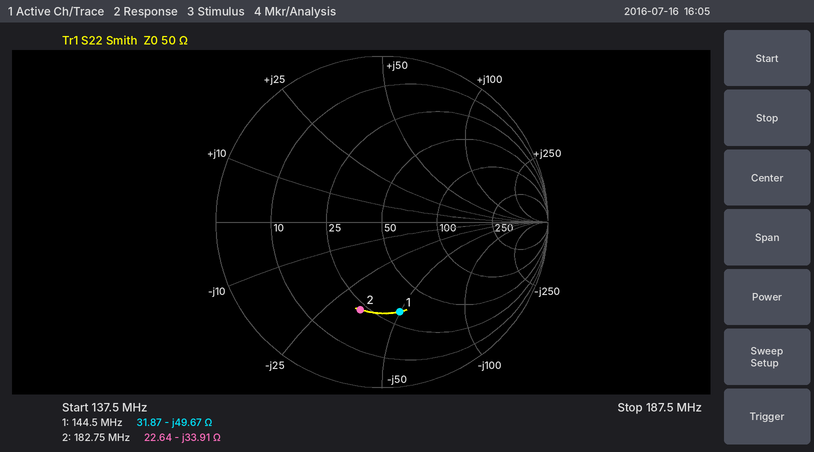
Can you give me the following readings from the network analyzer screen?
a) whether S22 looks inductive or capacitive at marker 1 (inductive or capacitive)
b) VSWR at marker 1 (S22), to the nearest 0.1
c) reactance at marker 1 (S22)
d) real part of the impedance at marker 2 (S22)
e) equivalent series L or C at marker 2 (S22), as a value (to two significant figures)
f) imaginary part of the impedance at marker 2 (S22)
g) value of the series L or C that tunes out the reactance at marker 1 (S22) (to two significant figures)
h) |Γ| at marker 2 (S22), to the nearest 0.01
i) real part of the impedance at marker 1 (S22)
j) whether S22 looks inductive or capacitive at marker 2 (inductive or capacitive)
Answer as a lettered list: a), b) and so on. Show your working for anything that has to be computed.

a) capacitive
b) 3.5
c) -49.67 Ω
d) 22.64 Ω
e) C = 1/(2π × 182.75 MHz × 33.91 Ω) ≈ 26 pF
f) -33.91 Ω
g) L = 49.67 Ω/(2π × 144.5 MHz) ≈ 55 nH
h) 0.54
i) 31.87 Ω
j) capacitive
